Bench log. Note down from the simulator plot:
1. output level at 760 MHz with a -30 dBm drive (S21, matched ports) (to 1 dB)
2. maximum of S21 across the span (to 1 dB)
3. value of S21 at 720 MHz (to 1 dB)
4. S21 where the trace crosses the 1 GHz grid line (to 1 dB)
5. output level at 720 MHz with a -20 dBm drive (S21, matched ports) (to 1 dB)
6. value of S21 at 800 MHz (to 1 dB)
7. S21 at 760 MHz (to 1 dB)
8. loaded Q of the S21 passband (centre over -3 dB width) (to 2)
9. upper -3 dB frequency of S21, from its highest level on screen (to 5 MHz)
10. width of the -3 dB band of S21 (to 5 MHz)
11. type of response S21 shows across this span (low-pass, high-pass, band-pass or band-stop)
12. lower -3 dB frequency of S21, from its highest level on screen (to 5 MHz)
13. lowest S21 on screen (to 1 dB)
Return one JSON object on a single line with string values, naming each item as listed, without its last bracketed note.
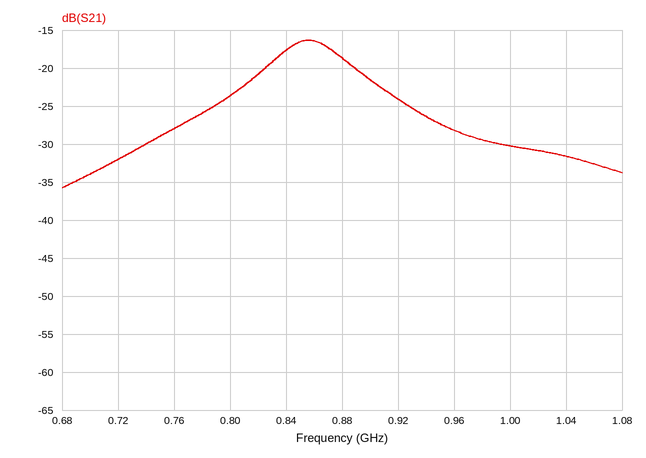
{"output level at 760 MHz with a -30 dBm drive (S21, matched ports)": "-58 dBm", "maximum of S21 across the span": "-16 dB", "value of S21 at 720 MHz": "-32 dB", "S21 where the trace crosses the 1 GHz grid line": "-30 dB", "output level at 720 MHz with a -20 dBm drive (S21, matched ports)": "-52 dBm", "value of S21 at 800 MHz": "-24 dB", "S21 at 760 MHz": "-28 dB", "loaded Q of the S21 passband (centre over -3 dB width)": "16", "upper -3 dB frequency of S21, from its highest level on screen": "885 MHz", "width of the -3 dB band of S21": "55 MHz", "type of response S21 shows across this span": "band-pass", "lower -3 dB frequency of S21, from its highest level on screen": "830 MHz", "lowest S21 on screen": "-36 dB"}
